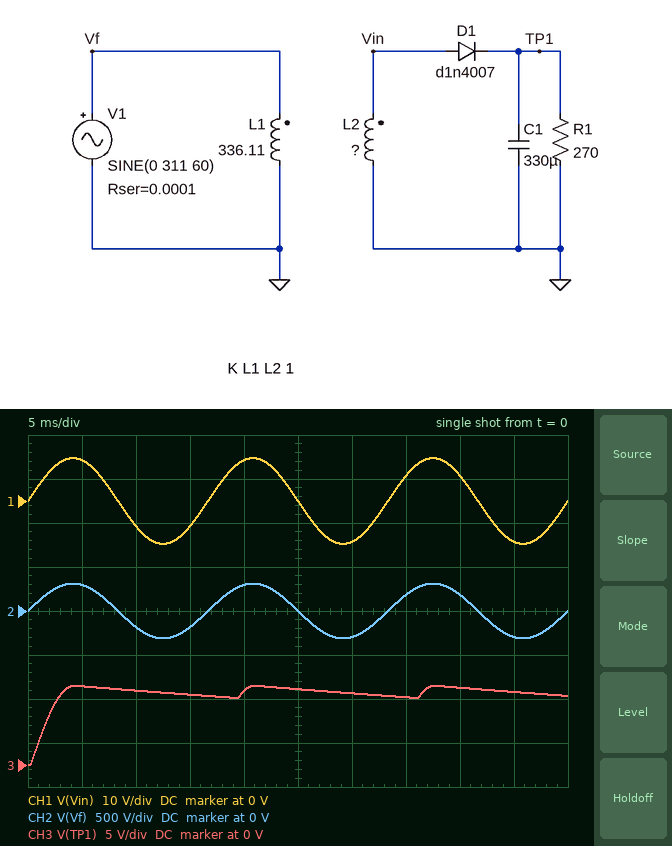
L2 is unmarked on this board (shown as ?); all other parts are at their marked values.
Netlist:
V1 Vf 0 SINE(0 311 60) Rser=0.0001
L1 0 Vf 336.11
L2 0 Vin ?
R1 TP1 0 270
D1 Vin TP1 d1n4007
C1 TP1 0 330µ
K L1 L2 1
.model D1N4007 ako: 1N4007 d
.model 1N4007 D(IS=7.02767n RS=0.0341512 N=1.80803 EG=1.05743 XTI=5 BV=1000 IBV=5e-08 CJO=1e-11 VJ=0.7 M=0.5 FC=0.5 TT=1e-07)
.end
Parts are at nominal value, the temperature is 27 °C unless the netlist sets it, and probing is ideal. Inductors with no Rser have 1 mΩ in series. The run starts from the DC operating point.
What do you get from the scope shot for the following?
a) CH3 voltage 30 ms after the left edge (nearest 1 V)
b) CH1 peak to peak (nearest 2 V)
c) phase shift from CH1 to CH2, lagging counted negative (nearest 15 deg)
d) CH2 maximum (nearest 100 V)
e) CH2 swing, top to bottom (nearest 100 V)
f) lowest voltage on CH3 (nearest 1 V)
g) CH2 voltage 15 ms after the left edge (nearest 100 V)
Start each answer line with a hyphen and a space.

- 8 V
- 20 V
- 0 deg
- 300 V
- 600 V
- 0 V
- -200 V
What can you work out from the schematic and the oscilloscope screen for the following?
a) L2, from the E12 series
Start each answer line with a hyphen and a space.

- 330 mH
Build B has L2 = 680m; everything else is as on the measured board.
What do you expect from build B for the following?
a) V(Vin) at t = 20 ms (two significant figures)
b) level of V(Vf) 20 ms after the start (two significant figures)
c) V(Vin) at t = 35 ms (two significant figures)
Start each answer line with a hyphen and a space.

- 13 V
- 300 V
- 8.2 V
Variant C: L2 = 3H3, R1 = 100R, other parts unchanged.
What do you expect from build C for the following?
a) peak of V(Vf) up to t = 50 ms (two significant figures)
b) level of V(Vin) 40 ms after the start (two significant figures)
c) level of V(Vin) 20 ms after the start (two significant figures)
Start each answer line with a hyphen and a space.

- 310 V
- 18 V
- 29 V
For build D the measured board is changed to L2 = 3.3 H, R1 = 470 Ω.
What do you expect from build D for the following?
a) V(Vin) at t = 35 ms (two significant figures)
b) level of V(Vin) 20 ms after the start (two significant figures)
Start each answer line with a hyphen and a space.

- 18 V
- 29 V
